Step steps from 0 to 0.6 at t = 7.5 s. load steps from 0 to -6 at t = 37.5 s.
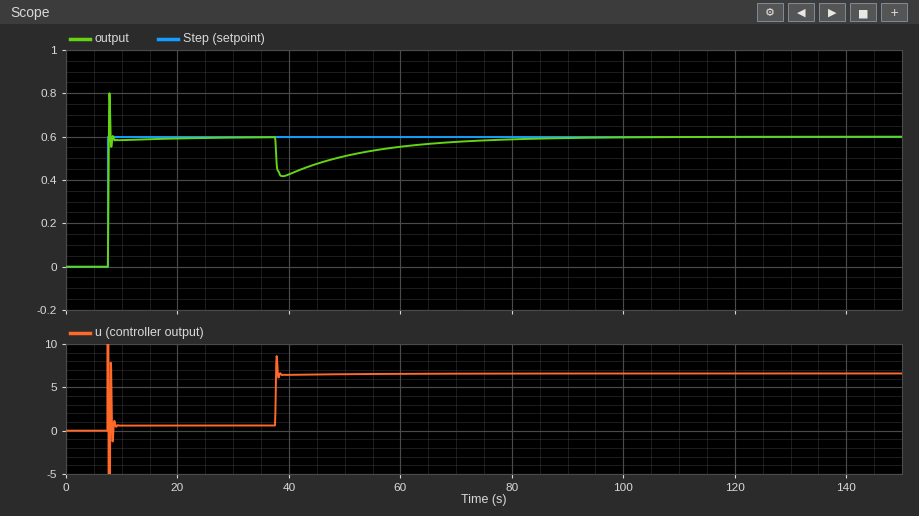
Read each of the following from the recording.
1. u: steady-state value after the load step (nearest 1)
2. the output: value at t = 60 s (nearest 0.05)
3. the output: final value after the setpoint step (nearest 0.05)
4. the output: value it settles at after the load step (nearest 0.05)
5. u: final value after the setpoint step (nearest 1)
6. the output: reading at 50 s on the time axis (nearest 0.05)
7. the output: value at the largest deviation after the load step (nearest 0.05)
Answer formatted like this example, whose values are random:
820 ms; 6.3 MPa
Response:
7; 0.55; 0.60; 0.60; 1; 0.50; 0.40
